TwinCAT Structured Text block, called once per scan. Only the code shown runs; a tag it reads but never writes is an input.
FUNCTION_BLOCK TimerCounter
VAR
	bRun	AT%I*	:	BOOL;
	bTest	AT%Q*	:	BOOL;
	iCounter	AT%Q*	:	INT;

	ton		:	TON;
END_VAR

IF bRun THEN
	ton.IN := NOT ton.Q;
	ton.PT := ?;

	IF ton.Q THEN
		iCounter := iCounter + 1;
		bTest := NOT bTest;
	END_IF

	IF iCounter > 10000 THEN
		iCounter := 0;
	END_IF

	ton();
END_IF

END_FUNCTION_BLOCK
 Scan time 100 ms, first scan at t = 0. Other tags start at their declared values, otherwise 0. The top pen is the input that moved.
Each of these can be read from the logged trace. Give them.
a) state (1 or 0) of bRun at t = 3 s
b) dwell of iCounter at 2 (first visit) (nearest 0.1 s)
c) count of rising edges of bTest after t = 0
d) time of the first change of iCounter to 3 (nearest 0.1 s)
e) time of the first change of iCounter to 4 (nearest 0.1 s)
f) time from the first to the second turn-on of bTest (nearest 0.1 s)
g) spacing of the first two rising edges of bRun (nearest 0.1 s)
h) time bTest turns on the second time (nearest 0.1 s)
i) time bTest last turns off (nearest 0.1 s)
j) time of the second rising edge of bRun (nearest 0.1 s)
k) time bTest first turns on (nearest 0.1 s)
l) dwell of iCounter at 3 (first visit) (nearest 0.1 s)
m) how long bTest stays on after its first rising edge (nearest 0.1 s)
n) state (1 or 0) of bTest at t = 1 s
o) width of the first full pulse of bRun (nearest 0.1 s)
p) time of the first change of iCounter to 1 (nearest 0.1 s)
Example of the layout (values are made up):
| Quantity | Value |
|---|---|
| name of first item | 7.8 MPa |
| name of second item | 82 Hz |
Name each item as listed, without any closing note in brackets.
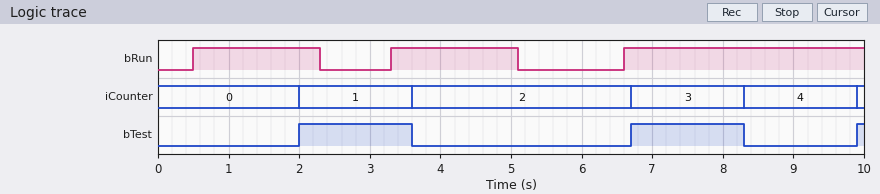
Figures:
| Quantity | Value |
|---|---|
| state (1 or 0) of bRun at t = 3 s | 0 |
| dwell of iCounter at 2 (first visit) | 3.1 s |
| count of rising edges of bTest after t = 0 | 3 |
| time of the first change of iCounter to 3 | 6.7 s |
| time of the first change of iCounter to 4 | 8.3 s |
| time from the first to the second turn-on of bTest | 4.7 s |
| spacing of the first two rising edges of bRun | 2.8 s |
| time bTest turns on the second time | 6.7 s |
| time bTest last turns off | 8.3 s |
| time of the second rising edge of bRun | 3.3 s |
| time bTest first turns on | 2.0 s |
| dwell of iCounter at 3 (first visit) | 1.6 s |
| how long bTest stays on after its first rising edge | 1.6 s |
| state (1 or 0) of bTest at t = 1 s | 0 |
| width of the first full pulse of bRun | 1.8 s |
| time of the first change of iCounter to 1 | 2.0 s |
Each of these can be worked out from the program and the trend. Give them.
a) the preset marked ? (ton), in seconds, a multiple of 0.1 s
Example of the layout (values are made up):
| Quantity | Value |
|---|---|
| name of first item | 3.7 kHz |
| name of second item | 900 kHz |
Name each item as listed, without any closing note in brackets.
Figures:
| Quantity | Value |
|---|---|
| the preset marked ? (ton), in seconds, a multiple of 0.1 s | 1.4 s |
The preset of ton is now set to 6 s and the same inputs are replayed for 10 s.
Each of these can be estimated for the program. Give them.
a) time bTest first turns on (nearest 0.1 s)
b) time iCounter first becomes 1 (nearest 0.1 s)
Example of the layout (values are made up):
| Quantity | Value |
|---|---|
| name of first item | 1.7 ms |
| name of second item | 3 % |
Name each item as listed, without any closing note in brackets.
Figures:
| Quantity | Value |
|---|---|
| time bTest first turns on | 6.7 s |
| time iCounter first becomes 1 | 6.7 s |
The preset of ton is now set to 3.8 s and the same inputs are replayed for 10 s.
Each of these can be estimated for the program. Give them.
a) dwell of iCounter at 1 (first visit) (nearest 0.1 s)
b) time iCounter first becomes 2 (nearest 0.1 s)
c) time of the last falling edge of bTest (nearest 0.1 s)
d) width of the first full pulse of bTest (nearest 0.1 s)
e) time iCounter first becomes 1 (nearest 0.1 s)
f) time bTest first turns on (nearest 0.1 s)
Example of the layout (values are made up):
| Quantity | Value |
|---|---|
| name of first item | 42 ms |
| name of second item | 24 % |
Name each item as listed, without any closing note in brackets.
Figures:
| Quantity | Value |
|---|---|
| dwell of iCounter at 1 (first visit) | 4.0 s |
| time iCounter first becomes 2 | 8.4 s |
| time of the last falling edge of bTest | 8.4 s |
| width of the first full pulse of bTest | 4.0 s |
| time iCounter first becomes 1 | 4.4 s |
| time bTest first turns on | 4.4 s |
